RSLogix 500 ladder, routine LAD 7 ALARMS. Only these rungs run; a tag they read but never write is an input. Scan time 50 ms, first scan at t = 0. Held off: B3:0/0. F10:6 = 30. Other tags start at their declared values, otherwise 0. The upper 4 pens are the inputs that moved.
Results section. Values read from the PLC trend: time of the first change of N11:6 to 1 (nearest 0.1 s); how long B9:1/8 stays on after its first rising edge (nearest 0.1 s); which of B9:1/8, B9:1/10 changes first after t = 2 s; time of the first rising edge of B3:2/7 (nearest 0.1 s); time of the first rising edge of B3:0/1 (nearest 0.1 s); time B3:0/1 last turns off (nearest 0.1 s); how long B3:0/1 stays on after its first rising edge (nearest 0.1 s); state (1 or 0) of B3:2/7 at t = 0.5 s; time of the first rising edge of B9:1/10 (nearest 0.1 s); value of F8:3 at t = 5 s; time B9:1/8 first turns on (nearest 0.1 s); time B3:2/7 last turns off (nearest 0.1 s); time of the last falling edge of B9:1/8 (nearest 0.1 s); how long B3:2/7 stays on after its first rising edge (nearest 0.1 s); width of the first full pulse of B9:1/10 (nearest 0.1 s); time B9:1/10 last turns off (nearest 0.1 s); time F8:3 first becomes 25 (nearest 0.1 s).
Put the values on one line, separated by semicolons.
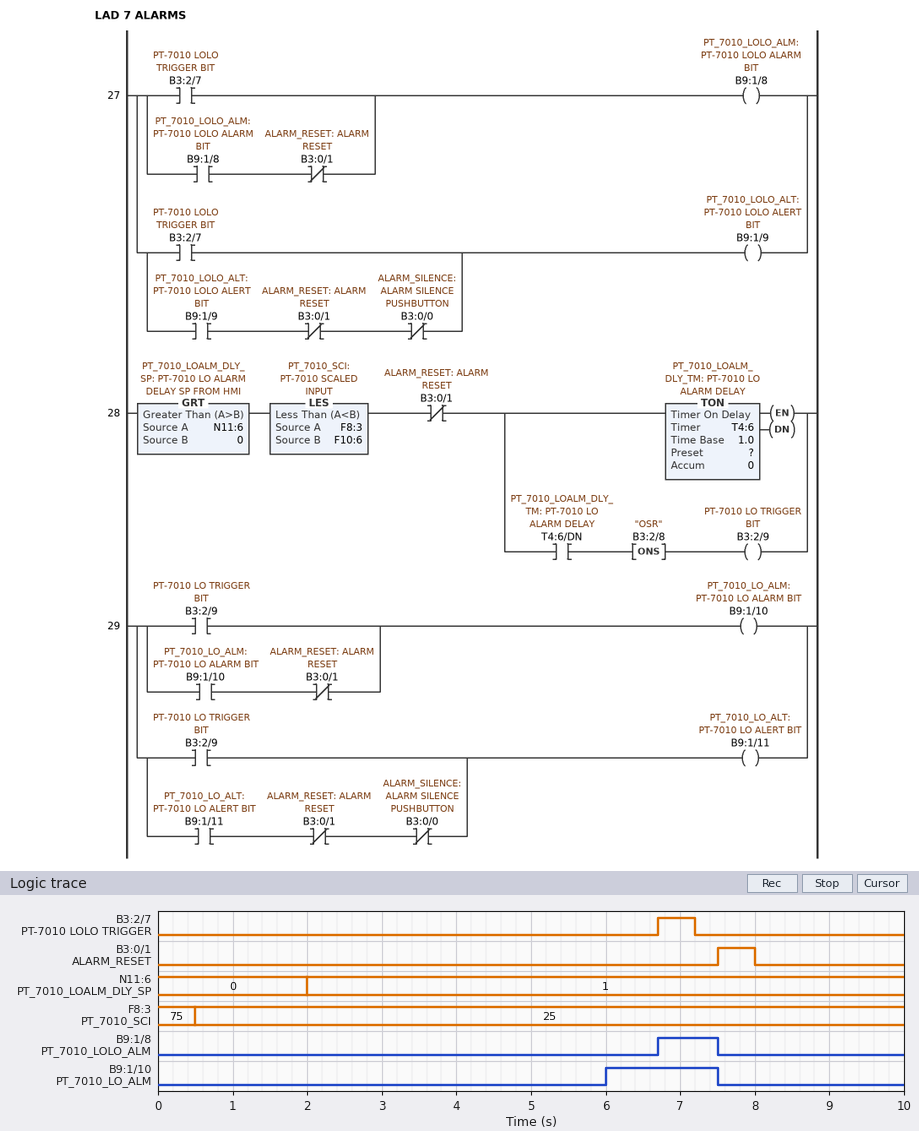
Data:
2.0 s; 0.8 s; B9:1/10; 6.7 s; 7.5 s; 8.0 s; 0.5 s; 0; 6.0 s; 25; 6.7 s; 7.2 s; 7.5 s; 0.5 s; 1.5 s; 7.5 s; 0.5 s
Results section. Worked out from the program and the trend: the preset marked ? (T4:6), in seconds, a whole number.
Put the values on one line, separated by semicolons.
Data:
4 s
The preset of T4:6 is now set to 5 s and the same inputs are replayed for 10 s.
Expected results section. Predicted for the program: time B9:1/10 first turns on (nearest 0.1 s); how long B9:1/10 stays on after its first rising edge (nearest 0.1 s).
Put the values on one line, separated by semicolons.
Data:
7.0 s; 0.5 s
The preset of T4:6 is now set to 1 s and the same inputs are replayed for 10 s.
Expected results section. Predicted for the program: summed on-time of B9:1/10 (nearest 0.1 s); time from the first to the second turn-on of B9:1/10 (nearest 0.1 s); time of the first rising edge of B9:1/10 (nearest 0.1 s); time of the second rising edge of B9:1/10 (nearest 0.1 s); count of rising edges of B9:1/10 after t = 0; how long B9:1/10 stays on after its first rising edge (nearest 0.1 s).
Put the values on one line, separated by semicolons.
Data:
5.5 s; 6.0 s; 3.0 s; 9.0 s; 2; 4.5 s
